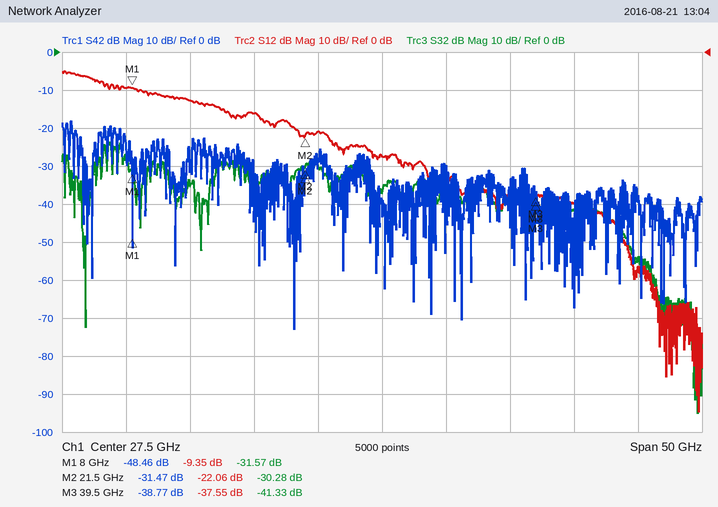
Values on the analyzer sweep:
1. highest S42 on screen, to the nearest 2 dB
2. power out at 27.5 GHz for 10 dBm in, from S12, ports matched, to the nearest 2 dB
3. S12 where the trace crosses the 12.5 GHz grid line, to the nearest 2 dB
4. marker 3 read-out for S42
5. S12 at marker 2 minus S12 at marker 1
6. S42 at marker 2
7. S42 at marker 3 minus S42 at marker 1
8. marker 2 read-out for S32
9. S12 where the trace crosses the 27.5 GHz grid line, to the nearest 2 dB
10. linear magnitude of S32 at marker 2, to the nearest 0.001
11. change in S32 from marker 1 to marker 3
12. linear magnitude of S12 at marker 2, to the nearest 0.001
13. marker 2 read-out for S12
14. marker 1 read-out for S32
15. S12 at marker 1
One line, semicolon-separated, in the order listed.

-18 dB; -18 dBm; -12 dB; -38.77 dB; -12.71 dB; -31.47 dB; 9.69 dB; -30.28 dB; -28 dB; 0.031; -9.76 dB; 0.079; -22.06 dB; -31.57 dB; -9.35 dB
